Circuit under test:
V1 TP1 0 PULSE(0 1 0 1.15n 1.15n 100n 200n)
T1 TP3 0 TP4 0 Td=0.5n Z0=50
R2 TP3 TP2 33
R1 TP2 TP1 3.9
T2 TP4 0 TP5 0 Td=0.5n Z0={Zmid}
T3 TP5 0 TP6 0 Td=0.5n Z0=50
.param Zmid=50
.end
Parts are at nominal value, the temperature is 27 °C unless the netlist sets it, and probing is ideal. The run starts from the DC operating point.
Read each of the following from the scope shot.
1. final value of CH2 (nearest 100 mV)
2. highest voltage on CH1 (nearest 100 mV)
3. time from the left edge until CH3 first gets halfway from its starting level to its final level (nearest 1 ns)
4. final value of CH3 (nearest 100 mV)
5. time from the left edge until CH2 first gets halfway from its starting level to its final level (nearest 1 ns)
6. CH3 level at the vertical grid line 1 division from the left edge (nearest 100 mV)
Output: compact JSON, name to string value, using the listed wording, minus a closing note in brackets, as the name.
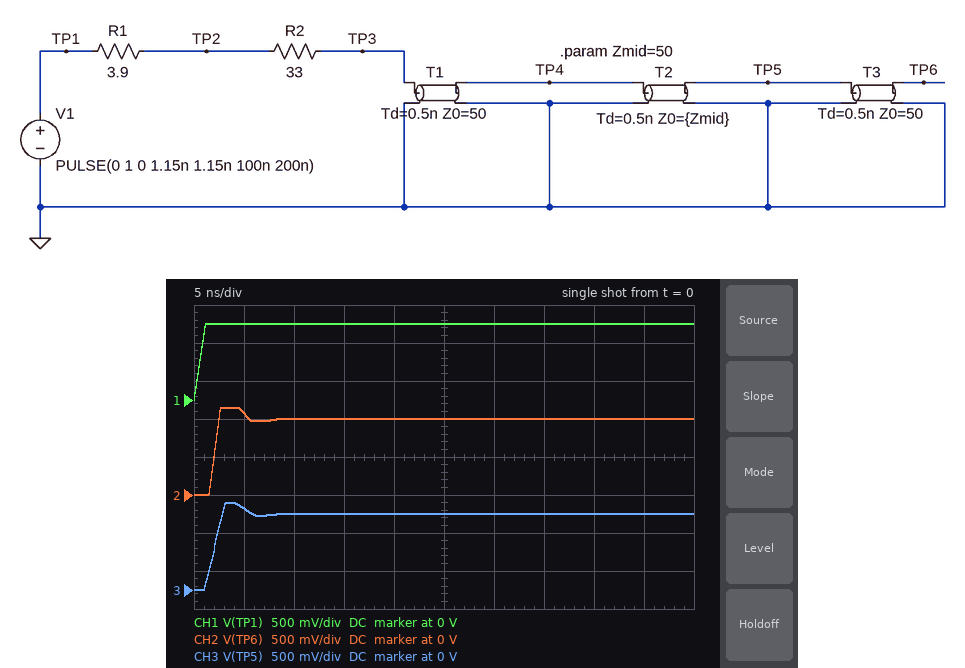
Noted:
{"final value of CH2": "1.0 V", "highest voltage on CH1": "1.0 V", "time from the left edge until CH3 first gets halfway from its starting level to its final level": "2 ns", "final value of CH3": "1.0 V", "time from the left edge until CH2 first gets halfway from its starting level to its final level": "2 ns", "CH3 level at the vertical grid line 1 division from the left edge": "1.1 V"}
